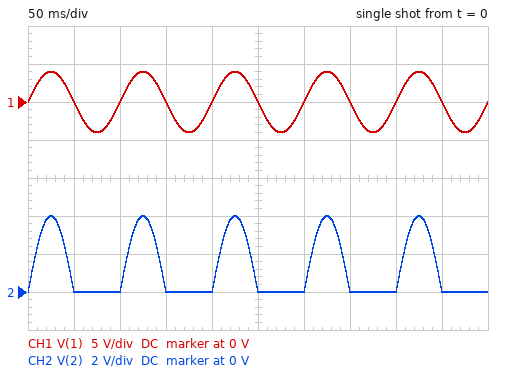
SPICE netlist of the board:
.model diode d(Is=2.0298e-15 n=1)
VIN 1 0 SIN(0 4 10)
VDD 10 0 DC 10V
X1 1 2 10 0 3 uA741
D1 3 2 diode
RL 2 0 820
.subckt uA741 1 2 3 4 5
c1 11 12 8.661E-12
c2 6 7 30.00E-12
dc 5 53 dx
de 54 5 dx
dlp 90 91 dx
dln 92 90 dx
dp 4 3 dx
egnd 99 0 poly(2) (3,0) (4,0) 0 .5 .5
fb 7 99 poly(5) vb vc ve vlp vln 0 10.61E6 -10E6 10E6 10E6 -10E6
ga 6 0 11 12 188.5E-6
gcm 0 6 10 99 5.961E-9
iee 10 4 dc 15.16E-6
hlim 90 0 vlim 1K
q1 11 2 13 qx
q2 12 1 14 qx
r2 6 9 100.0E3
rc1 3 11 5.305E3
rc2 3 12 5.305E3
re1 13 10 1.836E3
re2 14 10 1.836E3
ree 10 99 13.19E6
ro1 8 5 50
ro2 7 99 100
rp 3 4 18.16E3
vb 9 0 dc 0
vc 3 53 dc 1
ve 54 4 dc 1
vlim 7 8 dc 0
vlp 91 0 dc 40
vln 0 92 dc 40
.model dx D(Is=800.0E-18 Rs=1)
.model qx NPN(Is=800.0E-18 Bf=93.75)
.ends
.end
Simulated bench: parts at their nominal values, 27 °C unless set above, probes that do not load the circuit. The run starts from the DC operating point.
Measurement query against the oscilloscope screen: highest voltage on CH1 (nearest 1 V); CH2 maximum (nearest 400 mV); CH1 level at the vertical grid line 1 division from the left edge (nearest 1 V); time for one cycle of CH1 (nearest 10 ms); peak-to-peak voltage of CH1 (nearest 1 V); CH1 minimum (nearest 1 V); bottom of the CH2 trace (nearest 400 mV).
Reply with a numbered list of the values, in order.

1. 4 V
2. 4.0 V
3. 0 V
4. 100 ms
5. 8 V
6. -4 V
7. 0 V
